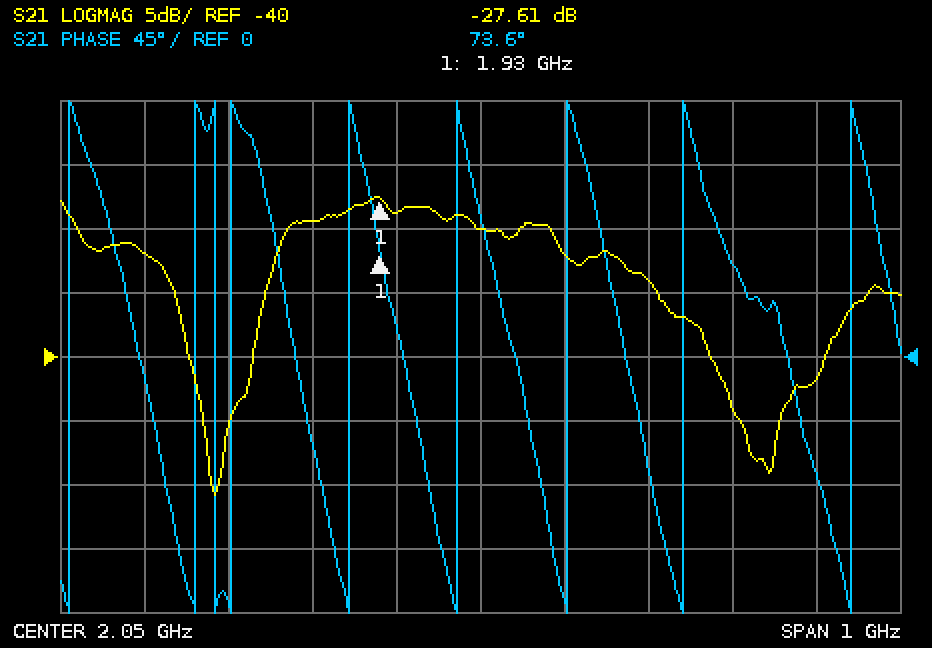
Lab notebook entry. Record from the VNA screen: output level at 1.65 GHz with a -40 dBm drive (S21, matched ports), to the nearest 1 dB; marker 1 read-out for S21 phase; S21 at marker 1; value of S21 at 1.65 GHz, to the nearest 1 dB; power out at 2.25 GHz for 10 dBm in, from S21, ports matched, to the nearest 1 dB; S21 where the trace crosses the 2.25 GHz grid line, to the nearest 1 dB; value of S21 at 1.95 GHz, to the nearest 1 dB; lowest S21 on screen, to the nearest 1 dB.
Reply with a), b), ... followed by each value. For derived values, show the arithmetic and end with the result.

a) -40 dBm + (-32 dB) = -72 dBm
b) 73.6°
c) -27.61 dB
d) -32 dB
e) 10 dBm + (-34 dB) = -24 dBm
f) -34 dB
g) -29 dB
h) -51 dB
